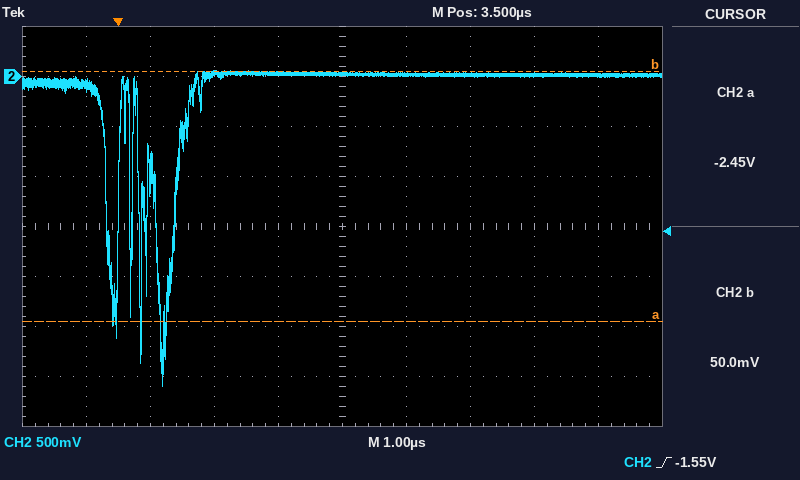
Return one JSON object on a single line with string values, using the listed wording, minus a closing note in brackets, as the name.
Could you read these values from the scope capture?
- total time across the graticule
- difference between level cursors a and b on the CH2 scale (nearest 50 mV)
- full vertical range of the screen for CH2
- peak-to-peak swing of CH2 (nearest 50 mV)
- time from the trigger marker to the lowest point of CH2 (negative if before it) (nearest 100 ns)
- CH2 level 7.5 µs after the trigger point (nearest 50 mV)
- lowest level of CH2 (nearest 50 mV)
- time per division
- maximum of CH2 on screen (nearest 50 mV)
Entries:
{"total time across the graticule": "10 µs", "difference between level cursors a and b on the CH2 scale": "2.50 V", "full vertical range of the screen for CH2": "4 V", "peak-to-peak swing of CH2": "3.15 V", "time from the trigger marker to the lowest point of CH2 (negative if before it)": "+700 ns", "CH2 level 7.5 µs after the trigger point": "0 mV", "lowest level of CH2": "-3.10 V", "time per division": "1 µs", "maximum of CH2 on screen": "50 mV"}
